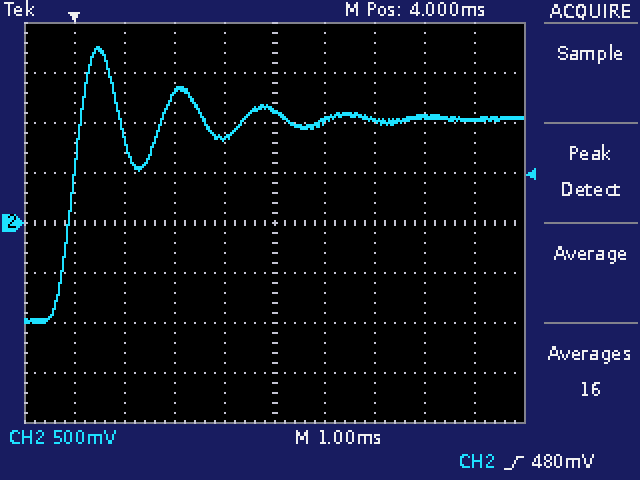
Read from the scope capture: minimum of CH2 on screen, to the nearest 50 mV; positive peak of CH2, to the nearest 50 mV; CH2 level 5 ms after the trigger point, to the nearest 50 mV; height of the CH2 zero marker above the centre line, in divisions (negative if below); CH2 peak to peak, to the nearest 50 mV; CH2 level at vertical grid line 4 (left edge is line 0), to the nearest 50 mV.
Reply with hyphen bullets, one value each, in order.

- -1.00 V
- 1.75 V
- 1.00 V
- 0.0 div
- 2.75 V
- 850 mV
